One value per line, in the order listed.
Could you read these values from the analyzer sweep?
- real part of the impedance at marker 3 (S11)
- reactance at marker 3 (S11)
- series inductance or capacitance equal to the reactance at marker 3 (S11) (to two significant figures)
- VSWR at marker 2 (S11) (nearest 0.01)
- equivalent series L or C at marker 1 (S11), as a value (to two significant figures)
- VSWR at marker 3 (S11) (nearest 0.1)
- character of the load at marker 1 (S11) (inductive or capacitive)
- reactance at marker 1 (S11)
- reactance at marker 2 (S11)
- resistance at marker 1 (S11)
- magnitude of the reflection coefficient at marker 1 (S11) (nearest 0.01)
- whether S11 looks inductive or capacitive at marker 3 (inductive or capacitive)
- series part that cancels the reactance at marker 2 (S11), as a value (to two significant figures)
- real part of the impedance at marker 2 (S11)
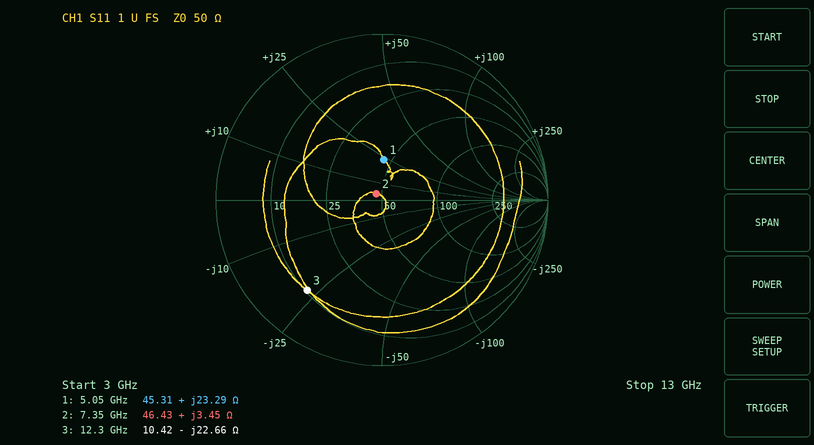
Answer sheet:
10.42 Ω
-22.66 Ω
570 fF
1.11
730 pH
5.8
inductive
+23.29 Ω
+3.45 Ω
45.31 Ω
0.24
capacitive
6.3 pF
46.43 Ω
